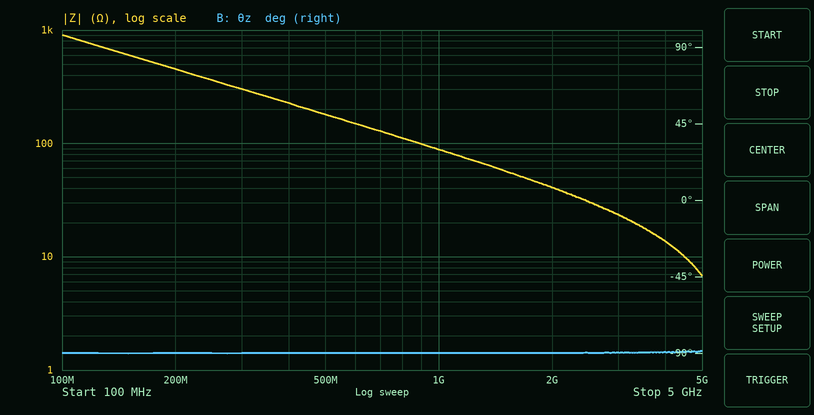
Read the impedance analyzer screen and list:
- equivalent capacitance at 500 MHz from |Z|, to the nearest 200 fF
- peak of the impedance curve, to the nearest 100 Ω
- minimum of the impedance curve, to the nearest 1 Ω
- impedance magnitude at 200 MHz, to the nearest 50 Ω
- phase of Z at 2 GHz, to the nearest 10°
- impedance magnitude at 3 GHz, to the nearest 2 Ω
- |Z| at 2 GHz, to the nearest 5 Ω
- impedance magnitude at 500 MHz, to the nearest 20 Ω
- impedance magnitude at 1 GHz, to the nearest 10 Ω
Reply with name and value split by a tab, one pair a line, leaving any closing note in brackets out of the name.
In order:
equivalent capacitance at 500 MHz from |Z|, to the nearest 200 fF	1.8 pF
peak of the impedance curve, to the nearest 100 Ω	900 Ω
minimum of the impedance curve, to the nearest 1 Ω	7 Ω
impedance magnitude at 200 MHz, to the nearest 50 Ω	450 Ω
phase of Z at 2 GHz, to the nearest 10°	-90°
impedance magnitude at 3 GHz, to the nearest 2 Ω	24 Ω
|Z| at 2 GHz, to the nearest 5 Ω	40 Ω
impedance magnitude at 500 MHz, to the nearest 20 Ω	180 Ω
impedance magnitude at 1 GHz, to the nearest 10 Ω	90 Ω
